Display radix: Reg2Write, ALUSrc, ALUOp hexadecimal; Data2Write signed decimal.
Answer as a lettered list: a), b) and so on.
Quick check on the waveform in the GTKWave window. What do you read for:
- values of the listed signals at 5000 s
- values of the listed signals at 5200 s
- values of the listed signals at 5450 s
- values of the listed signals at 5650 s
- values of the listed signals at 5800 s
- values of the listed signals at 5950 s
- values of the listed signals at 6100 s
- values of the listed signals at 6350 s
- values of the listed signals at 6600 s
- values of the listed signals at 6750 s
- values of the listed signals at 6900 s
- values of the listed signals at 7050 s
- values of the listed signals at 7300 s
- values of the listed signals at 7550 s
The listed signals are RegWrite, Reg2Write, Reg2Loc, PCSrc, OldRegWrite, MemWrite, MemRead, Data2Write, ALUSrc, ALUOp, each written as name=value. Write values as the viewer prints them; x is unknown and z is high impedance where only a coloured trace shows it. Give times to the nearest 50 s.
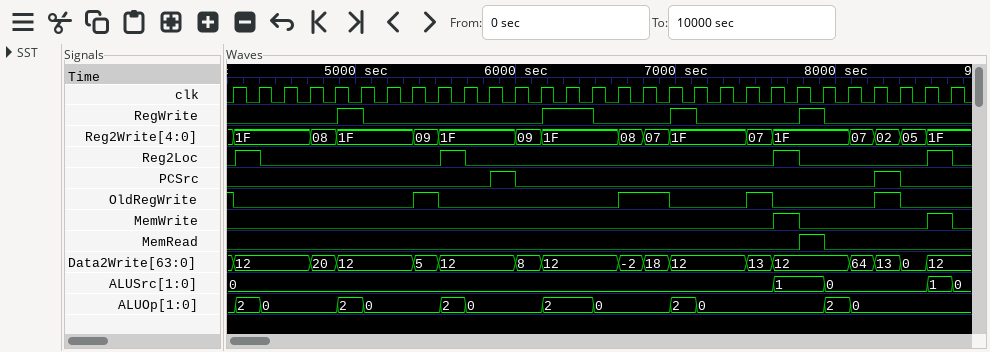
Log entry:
a) RegWrite=1, Reg2Write=1F, Reg2Loc=0, PCSrc=0, OldRegWrite=0, MemWrite=0, MemRead=0, Data2Write=12, ALUSrc=0, ALUOp=2
b) RegWrite=0, Reg2Write=1F, Reg2Loc=0, PCSrc=0, OldRegWrite=0, MemWrite=0, MemRead=0, Data2Write=12, ALUSrc=0, ALUOp=0
c) RegWrite=0, Reg2Write=09, Reg2Loc=0, PCSrc=0, OldRegWrite=1, MemWrite=0, MemRead=0, Data2Write=5, ALUSrc=0, ALUOp=0
d) RegWrite=0, Reg2Write=1F, Reg2Loc=1, PCSrc=0, OldRegWrite=0, MemWrite=0, MemRead=0, Data2Write=12, ALUSrc=0, ALUOp=2
e) RegWrite=0, Reg2Write=1F, Reg2Loc=0, PCSrc=0, OldRegWrite=0, MemWrite=0, MemRead=0, Data2Write=12, ALUSrc=0, ALUOp=0
f) RegWrite=0, Reg2Write=1F, Reg2Loc=0, PCSrc=1, OldRegWrite=0, MemWrite=0, MemRead=0, Data2Write=12, ALUSrc=0, ALUOp=0
g) RegWrite=0, Reg2Write=09, Reg2Loc=0, PCSrc=0, OldRegWrite=0, MemWrite=0, MemRead=0, Data2Write=8, ALUSrc=0, ALUOp=0
h) RegWrite=1, Reg2Write=1F, Reg2Loc=0, PCSrc=0, OldRegWrite=0, MemWrite=0, MemRead=0, Data2Write=12, ALUSrc=0, ALUOp=2
i) RegWrite=0, Reg2Write=1F, Reg2Loc=0, PCSrc=0, OldRegWrite=0, MemWrite=0, MemRead=0, Data2Write=12, ALUSrc=0, ALUOp=0
j) RegWrite=0, Reg2Write=08, Reg2Loc=0, PCSrc=0, OldRegWrite=1, MemWrite=0, MemRead=0, Data2Write=-2, ALUSrc=0, ALUOp=0
k) RegWrite=0, Reg2Write=07, Reg2Loc=0, PCSrc=0, OldRegWrite=1, MemWrite=0, MemRead=0, Data2Write=18, ALUSrc=0, ALUOp=0
l) RegWrite=1, Reg2Write=1F, Reg2Loc=0, PCSrc=0, OldRegWrite=0, MemWrite=0, MemRead=0, Data2Write=12, ALUSrc=0, ALUOp=2
m) RegWrite=0, Reg2Write=1F, Reg2Loc=0, PCSrc=0, OldRegWrite=0, MemWrite=0, MemRead=0, Data2Write=12, ALUSrc=0, ALUOp=0
n) RegWrite=0, Reg2Write=07, Reg2Loc=0, PCSrc=0, OldRegWrite=1, MemWrite=0, MemRead=0, Data2Write=13, ALUSrc=0, ALUOp=0
